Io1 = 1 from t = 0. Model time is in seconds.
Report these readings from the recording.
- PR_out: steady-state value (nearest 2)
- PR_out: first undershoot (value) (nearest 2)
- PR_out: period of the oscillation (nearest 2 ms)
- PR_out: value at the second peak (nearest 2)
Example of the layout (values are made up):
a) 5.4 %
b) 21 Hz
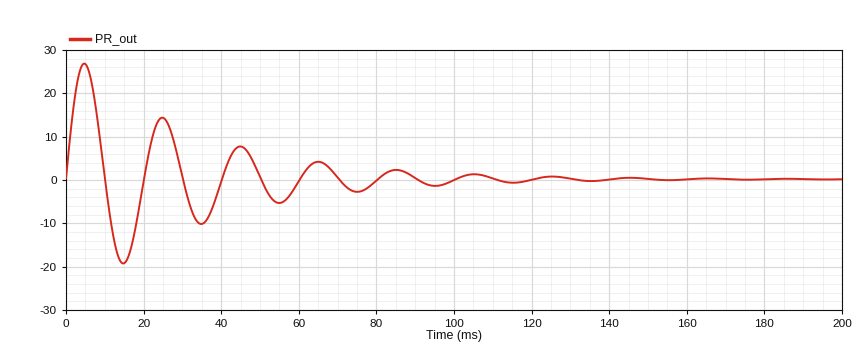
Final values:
a) 0
b) -20
c) 20 ms
d) 14
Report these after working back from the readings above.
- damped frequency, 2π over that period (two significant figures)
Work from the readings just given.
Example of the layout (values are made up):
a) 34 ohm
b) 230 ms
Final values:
a) 0.31 rad/ms
